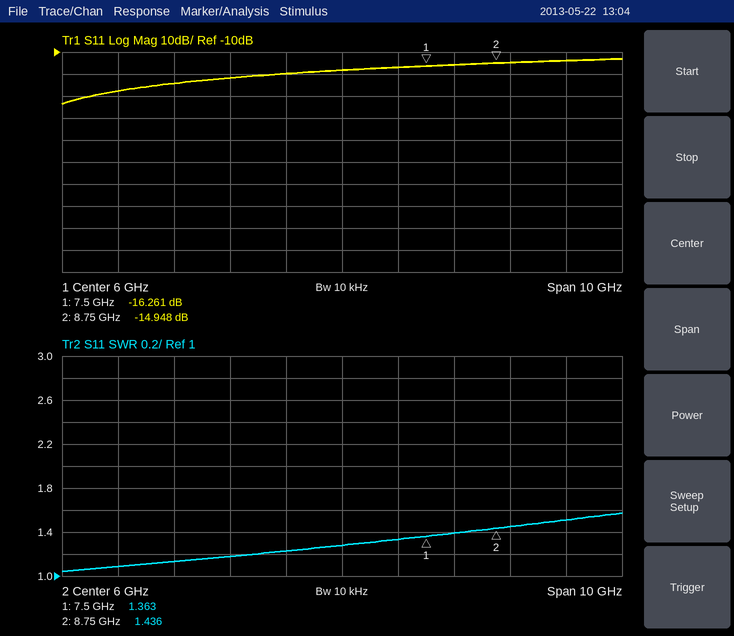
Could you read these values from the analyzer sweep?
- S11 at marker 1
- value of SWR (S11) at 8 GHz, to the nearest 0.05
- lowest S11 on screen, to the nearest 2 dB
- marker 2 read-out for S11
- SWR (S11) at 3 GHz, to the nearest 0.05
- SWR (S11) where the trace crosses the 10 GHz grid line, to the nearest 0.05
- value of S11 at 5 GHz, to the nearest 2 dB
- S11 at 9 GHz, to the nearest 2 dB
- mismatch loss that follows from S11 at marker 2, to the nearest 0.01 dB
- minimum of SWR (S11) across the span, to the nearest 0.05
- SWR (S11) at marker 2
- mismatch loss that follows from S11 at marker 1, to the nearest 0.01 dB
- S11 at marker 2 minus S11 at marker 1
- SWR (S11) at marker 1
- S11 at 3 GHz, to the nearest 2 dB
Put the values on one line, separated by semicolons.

-16.261 dB; 1.40; -34 dB; -14.948 dB; 1.15; 1.50; -20 dB; -14 dB; 0.14 dB; 1.05; 1.436; 0.10 dB; 1.313 dB; 1.363; -24 dB
